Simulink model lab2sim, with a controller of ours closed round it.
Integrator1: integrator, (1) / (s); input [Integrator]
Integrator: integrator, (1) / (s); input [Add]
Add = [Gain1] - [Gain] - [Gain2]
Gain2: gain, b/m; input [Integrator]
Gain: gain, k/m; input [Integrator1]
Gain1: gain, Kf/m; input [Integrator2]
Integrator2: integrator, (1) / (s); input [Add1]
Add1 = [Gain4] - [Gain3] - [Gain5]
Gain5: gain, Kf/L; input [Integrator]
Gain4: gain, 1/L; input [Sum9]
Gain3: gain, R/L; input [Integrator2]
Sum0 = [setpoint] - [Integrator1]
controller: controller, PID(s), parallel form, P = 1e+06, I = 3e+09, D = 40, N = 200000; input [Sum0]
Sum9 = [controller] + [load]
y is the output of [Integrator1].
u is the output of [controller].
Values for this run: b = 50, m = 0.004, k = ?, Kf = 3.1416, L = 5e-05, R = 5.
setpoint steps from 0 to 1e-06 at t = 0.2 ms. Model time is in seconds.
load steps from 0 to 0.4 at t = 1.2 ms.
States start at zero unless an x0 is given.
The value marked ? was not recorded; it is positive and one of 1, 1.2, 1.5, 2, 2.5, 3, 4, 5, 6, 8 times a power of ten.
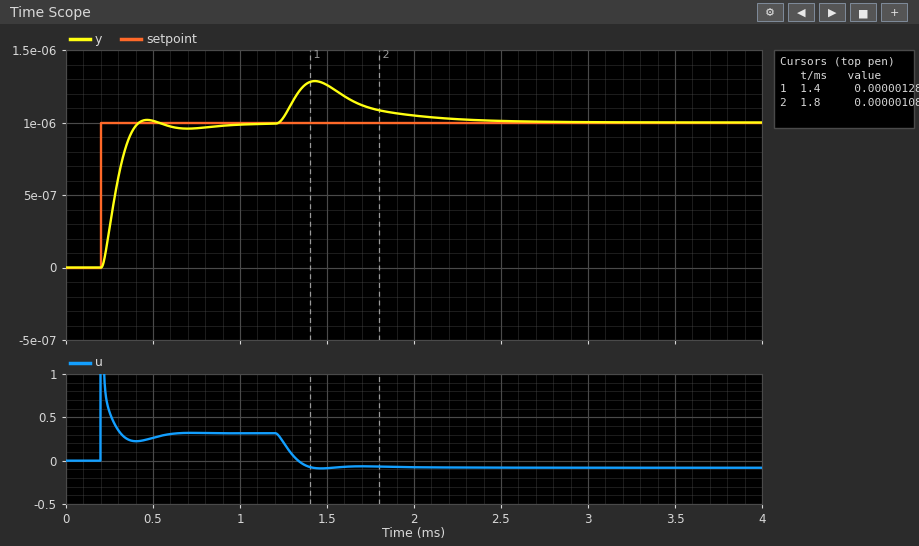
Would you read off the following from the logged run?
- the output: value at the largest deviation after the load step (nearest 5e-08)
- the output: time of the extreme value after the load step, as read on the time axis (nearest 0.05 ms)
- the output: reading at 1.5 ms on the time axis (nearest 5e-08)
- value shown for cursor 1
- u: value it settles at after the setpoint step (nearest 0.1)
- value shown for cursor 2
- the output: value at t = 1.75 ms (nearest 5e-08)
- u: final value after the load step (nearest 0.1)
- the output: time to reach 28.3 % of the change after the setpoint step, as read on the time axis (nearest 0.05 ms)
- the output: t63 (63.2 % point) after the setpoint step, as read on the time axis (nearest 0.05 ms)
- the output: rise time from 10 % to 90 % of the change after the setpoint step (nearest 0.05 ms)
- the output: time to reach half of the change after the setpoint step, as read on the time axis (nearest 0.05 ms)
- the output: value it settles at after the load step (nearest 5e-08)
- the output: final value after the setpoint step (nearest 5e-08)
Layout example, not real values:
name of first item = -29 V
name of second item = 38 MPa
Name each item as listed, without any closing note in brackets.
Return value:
the output: value at the largest deviation after the load step = 0.00000130
the output: time of the extreme value after the load step, as read on the time axis = 1.45 ms
the output: reading at 1.5 ms on the time axis = 0.00000125
value shown for cursor 1 = 0.000001280
u: value it settles at after the setpoint step = 0.3
value shown for cursor 2 = 0.000001085
the output: value at t = 1.75 ms = 0.00000110
u: final value after the load step = -0.1
the output: time to reach 28.3 % of the change after the setpoint step, as read on the time axis = 0.25 ms
the output: t63 (63.2 % point) after the setpoint step, as read on the time axis = 0.30 ms
the output: rise time from 10 % to 90 % of the change after the setpoint step = 0.15 ms
the output: time to reach half of the change after the setpoint step, as read on the time axis = 0.30 ms
the output: value it settles at after the load step = 0.00000100
the output: final value after the setpoint step = 0.00000100
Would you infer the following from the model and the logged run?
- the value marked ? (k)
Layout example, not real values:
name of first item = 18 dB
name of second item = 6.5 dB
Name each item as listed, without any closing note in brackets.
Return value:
the value marked ? = 200000
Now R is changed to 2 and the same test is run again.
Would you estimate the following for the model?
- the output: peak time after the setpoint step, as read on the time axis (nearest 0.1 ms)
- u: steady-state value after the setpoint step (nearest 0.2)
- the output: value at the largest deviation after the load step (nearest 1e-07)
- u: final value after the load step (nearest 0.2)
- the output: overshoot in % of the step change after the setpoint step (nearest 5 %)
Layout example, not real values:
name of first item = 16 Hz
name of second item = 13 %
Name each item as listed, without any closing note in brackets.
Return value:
the output: peak time after the setpoint step, as read on the time axis = 0.3 ms
u: steady-state value after the setpoint step = 0.2
the output: value at the largest deviation after the load step = 0.0000014
u: final value after the load step = -0.2
the output: overshoot in % of the step change after the setpoint step = 25 %
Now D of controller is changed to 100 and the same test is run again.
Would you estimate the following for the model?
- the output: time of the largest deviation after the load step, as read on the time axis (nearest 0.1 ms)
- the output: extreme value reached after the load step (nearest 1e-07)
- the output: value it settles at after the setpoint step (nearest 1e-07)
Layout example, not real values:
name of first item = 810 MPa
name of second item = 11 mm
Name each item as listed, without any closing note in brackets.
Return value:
the output: time of the largest deviation after the load step, as read on the time axis = 1.5 ms
the output: extreme value reached after the load step = 0.0000012
the output: value it settles at after the setpoint step = 0.0000010
